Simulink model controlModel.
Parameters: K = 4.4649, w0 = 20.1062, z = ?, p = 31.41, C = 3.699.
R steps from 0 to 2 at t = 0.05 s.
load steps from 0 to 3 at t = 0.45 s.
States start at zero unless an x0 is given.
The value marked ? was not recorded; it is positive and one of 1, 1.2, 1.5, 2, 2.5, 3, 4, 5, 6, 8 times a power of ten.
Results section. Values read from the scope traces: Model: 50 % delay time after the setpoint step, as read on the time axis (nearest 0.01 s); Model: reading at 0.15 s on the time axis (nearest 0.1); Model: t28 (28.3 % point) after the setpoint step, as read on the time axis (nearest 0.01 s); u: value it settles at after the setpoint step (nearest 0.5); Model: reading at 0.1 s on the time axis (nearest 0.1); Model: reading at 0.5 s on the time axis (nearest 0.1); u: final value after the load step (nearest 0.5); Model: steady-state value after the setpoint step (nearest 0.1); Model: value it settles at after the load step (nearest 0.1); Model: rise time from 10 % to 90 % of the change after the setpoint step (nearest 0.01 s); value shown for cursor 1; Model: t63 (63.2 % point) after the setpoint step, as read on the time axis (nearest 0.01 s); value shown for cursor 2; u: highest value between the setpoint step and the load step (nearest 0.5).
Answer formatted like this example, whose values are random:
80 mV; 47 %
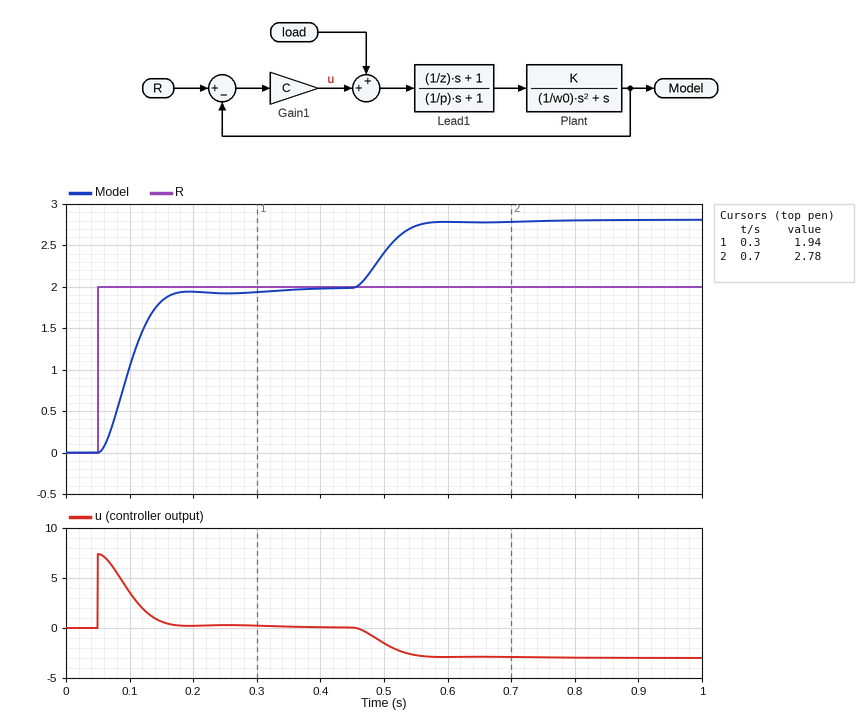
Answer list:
0.10 s; 1.8; 0.08 s; 0.0; 1.0; 2.4; -3.0; 2.0; 2.8; 0.08 s; 1.94; 0.11 s; 2.78; 7.5
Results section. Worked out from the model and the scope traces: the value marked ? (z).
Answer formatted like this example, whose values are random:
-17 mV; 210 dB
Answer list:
12
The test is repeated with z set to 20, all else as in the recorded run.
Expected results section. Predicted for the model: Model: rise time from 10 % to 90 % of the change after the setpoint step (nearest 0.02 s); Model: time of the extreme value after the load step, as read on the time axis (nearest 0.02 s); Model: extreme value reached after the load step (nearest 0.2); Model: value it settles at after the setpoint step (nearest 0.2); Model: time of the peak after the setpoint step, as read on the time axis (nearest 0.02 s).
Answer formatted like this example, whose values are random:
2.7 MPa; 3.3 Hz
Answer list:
0.10 s; 0.64 s; 2.8; 2.0; 0.24 s
